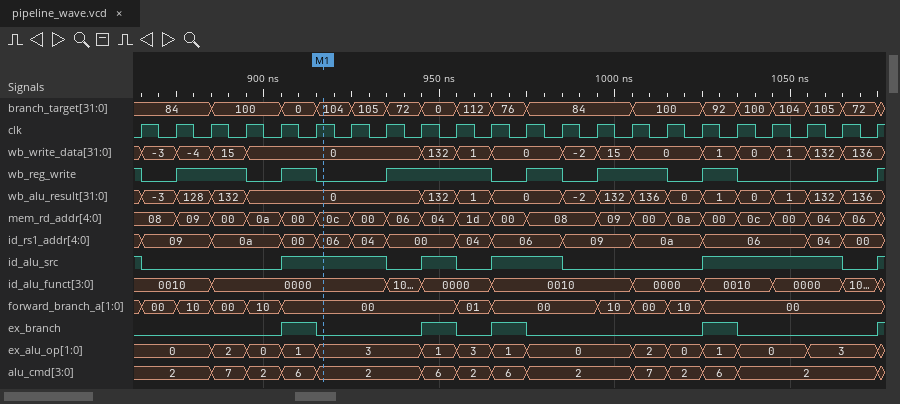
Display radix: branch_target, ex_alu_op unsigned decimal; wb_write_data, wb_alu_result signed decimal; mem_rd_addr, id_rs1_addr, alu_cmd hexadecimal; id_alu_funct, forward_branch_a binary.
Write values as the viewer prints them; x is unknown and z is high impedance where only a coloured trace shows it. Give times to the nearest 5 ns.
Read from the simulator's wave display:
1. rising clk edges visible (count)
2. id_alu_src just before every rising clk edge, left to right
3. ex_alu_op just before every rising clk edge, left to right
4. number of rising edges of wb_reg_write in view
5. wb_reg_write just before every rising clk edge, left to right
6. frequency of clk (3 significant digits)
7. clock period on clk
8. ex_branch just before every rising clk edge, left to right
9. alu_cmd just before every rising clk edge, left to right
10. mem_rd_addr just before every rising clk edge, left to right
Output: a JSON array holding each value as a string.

["22", "1 0 0 0 0 1 1 1 0 1 0 1 1 0 0 0 0 1 1 1 1 0", "0, 0, 0, 2, 0, 1, 3, 3, 3, 1, 3, 1, 0, 0, 0, 2, 0, 1, 0, 0, 3, 3", "7", "1 0 1 1 0 1 0 0 1 1 1 0 1 0 1 1 0 1 0 0 0 0", "100 MHz", "10 ns", "0 0 0 0 0 1 0 0 0 1 0 1 0 0 0 0 0 1 0 0 0 0", "2, 2, 2, 7, 2, 6, 2, 2, 2, 6, 2, 6, 2, 2, 2, 7, 2, 6, 2, 2, 2, 2", "08, 08, 09, 00, 0a, 00, 0c, 00, 06, 04, 1d, 00, 08, 08, 09, 00, 0a, 00, 0c, 00, 04, 06"]
